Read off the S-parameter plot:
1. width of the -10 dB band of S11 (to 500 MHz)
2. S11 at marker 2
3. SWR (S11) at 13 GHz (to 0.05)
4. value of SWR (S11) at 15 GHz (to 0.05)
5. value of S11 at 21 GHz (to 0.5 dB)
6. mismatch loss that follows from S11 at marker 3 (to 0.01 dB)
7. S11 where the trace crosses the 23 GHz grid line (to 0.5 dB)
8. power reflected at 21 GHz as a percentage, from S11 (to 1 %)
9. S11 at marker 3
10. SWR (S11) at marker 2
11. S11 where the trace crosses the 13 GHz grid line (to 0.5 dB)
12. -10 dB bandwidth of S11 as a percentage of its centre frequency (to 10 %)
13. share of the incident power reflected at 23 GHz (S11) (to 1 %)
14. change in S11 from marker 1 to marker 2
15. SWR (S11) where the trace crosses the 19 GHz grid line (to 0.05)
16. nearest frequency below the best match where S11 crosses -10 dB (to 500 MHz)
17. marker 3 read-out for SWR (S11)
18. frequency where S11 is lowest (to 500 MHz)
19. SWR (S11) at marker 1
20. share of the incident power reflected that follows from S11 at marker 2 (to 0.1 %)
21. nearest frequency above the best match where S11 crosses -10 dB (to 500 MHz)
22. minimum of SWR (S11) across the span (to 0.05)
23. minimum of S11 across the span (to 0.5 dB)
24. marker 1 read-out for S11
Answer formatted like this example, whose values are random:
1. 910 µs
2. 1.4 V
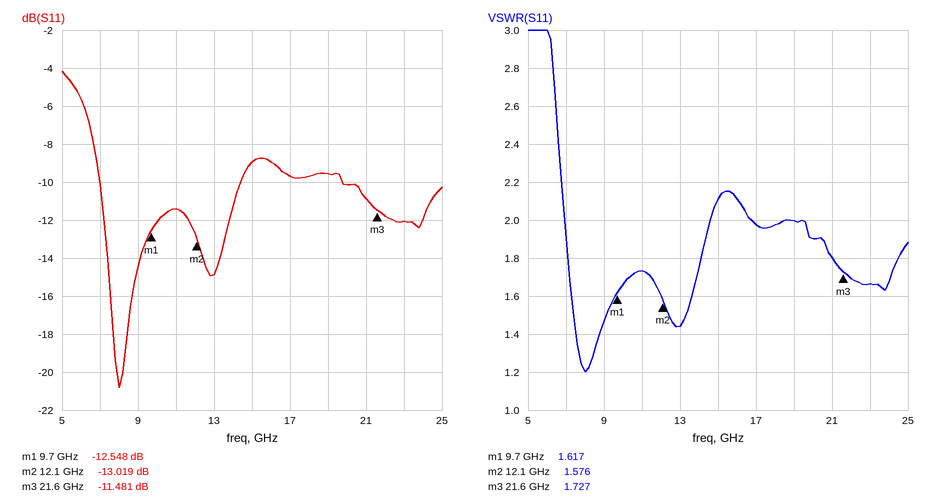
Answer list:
1. 7.5 GHz
2. -13.019 dB
3. 1.45
4. 2.10
5. -11.0 dB
6. 0.32 dB
7. -12.0 dB
8. 8 %
9. -11.481 dB
10. 1.576
11. -15.0 dB
12. 70 %
13. 6 %
14. -0.471 dB
15. 2.00
16. 7.0 GHz
17. 1.727
18. 8.0 GHz
19. 1.617
20. 5.0 %
21. 14.5 GHz
22. 1.20
23. -21.0 dB
24. -12.548 dB
